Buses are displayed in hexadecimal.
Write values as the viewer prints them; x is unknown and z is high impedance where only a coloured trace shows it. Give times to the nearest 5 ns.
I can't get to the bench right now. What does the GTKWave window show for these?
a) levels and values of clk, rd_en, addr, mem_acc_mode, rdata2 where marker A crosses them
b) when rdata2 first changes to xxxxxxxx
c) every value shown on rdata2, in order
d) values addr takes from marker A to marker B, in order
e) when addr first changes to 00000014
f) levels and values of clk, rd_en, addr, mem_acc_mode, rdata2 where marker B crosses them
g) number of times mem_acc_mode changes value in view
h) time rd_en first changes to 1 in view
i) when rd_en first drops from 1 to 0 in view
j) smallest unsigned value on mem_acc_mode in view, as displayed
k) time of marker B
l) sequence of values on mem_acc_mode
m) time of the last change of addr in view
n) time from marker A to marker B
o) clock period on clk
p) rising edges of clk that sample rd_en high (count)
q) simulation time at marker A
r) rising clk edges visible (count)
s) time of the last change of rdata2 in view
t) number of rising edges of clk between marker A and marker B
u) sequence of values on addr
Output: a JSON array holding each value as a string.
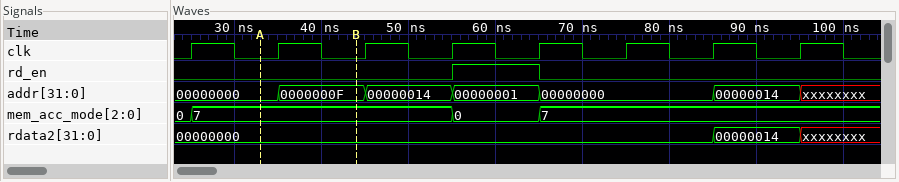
["clk=0, rd_en=0, addr=00000000, mem_acc_mode=7, rdata2=00000000", "95 ns", "00000000, 00000014, xxxxxxxx", "00000000, 0000000F", "45 ns", "clk=0, rd_en=0, addr=0000000F, mem_acc_mode=7, rdata2=00000000", "3", "55 ns", "65 ns", "0", "45 ns", "0, 7, 0, 7", "95 ns", "10 ns", "10 ns", "1", "35 ns", "8", "95 ns", "1", "00000000, 0000000F, 00000014, 00000001, 00000000, 00000014, xxxxxxxx"]
